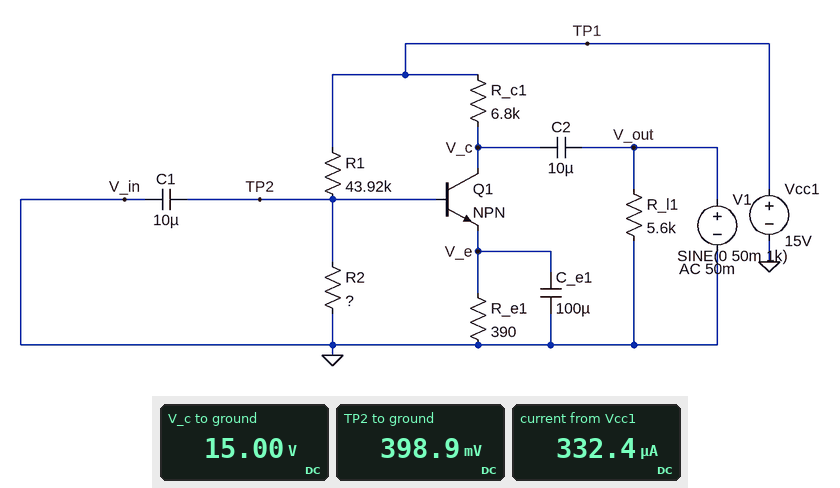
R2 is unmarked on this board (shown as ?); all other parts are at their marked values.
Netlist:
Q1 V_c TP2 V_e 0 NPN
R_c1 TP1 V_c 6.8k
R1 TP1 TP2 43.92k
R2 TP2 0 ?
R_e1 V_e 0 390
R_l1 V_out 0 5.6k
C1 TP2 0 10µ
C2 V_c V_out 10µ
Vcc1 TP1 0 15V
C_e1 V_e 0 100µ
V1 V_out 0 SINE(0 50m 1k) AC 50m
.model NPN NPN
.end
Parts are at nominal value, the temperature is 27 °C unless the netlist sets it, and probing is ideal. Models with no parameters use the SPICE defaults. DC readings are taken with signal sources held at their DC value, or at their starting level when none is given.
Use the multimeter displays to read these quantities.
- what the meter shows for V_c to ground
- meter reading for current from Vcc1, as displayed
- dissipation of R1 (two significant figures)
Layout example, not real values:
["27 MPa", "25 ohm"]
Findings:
["15.00 V", "332.4 µA", "4.9 mW"]
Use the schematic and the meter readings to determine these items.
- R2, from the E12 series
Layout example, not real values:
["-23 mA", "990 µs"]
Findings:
["1.2 kΩ"]
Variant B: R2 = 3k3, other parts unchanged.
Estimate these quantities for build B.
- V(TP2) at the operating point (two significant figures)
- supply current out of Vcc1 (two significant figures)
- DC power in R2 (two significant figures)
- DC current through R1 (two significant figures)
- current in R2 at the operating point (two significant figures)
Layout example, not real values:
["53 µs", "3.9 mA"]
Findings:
["1.0 V", "990 µA", "320 µW", "320 µA", "310 µA"]
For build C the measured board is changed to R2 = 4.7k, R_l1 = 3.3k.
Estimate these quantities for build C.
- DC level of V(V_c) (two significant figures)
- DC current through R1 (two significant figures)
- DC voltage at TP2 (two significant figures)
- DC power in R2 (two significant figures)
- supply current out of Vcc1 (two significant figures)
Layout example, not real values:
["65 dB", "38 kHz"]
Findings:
["4.6 V", "310 µA", "1.4 V", "410 µW", "1.8 mA"]
